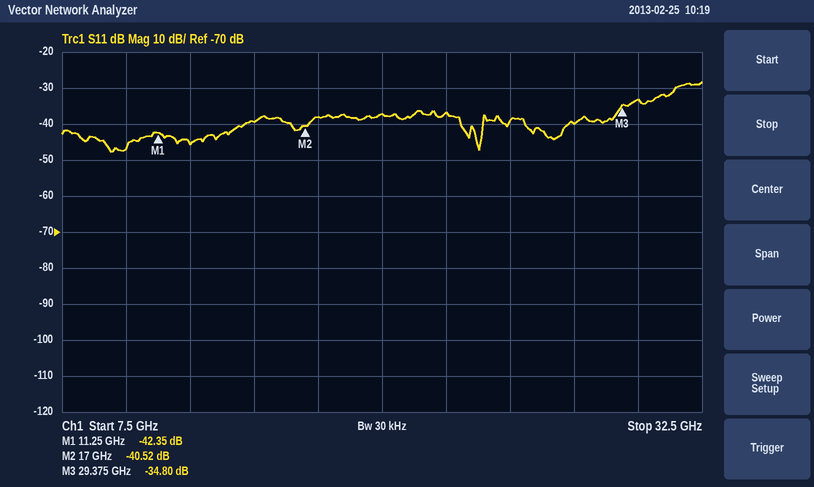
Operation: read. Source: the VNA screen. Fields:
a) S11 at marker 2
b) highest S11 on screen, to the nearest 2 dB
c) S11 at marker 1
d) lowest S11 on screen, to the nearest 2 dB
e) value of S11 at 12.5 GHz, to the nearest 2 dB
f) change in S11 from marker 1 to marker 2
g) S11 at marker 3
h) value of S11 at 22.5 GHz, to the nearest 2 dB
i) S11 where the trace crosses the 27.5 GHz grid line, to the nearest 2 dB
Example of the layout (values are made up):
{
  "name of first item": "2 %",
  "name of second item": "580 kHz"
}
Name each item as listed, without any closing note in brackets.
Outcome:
{
  "S11 at marker 2": "-40.52 dB",
  "highest S11 on screen, to the nearest 2 dB": "-28 dB",
  "S11 at marker 1": "-42.35 dB",
  "lowest S11 on screen, to the nearest 2 dB": "-48 dB",
  "value of S11 at 12.5 GHz, to the nearest 2 dB": "-46 dB",
  "change in S11 from marker 1 to marker 2": "1.83 dB",
  "S11 at marker 3": "-34.80 dB",
  "value of S11 at 22.5 GHz, to the nearest 2 dB": "-36 dB",
  "S11 where the trace crosses the 27.5 GHz grid line, to the nearest 2 dB": "-40 dB"
}
